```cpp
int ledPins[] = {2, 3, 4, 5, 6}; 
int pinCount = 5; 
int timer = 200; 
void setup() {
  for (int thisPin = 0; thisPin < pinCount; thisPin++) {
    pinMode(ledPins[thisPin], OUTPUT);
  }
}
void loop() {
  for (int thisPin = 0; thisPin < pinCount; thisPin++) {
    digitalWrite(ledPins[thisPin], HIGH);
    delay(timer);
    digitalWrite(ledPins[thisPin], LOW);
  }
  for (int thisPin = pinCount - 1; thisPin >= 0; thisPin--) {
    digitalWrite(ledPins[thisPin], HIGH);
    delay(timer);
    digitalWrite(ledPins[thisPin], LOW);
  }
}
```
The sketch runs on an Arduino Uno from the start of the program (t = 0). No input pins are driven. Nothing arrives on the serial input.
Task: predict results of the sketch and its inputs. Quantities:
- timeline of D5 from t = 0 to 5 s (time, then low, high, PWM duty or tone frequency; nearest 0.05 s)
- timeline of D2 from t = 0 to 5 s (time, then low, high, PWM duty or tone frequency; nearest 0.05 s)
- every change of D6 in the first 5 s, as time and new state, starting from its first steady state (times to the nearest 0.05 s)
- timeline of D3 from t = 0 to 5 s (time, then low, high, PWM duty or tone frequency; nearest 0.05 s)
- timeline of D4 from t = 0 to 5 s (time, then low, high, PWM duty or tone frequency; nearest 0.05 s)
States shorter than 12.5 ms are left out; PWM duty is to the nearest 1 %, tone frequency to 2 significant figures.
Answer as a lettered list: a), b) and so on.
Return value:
a) 0 s low; 0.6 s high; 0.8 s low; 1.2 s high; 1.4 s low; 2.6 s high; 2.8 s low; 3.2 s high; 3.4 s low; 4.6 s high; 4.8 s low
b) 0 s high; 0.2 s low; 1.8 s high; 2.2 s low; 3.8 s high; 4.2 s low
c) 0 s low; 0.8 s high; 1.2 s low; 2.8 s high; 3.2 s low; 4.8 s high
d) 0 s low; 0.2 s high; 0.4 s low; 1.6 s high; 1.8 s low; 2.2 s high; 2.4 s low; 3.6 s high; 3.8 s low; 4.2 s high; 4.4 s low
e) 0 s low; 0.4 s high; 0.6 s low; 1.4 s high; 1.6 s low; 2.4 s high; 2.6 s low; 3.4 s high; 3.6 s low; 4.4 s high; 4.6 s low
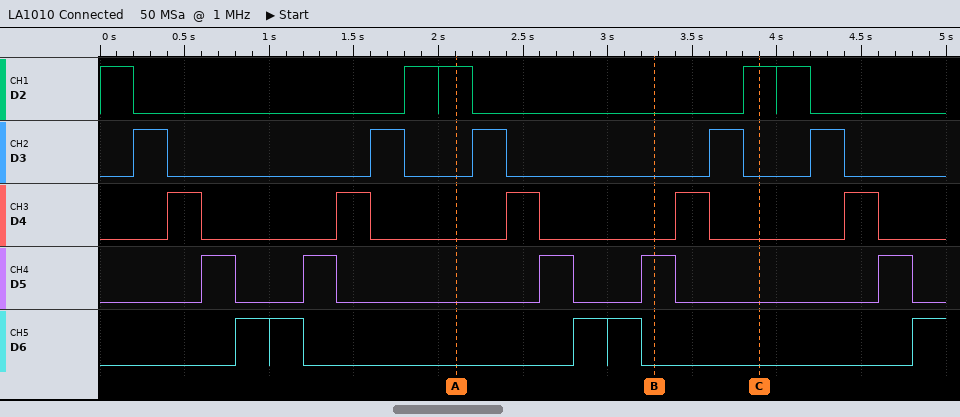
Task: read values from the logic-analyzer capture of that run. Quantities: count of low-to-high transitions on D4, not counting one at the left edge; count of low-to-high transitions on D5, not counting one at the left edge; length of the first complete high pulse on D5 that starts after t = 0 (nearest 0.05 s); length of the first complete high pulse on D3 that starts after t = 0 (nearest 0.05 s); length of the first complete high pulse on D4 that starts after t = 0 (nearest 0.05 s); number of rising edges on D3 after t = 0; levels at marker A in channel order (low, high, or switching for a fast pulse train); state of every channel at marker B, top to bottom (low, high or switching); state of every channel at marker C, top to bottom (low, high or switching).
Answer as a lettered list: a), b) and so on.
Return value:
a) 5
b) 5
c) 0.20 s
d) 0.20 s
e) 0.20 s
f) 5
g) D2 high, D3 low, D4 low, D5 low, D6 low
h) D2 low, D3 low, D4 low, D5 high, D6 low
i) D2 high, D3 low, D4 low, D5 low, D6 low
